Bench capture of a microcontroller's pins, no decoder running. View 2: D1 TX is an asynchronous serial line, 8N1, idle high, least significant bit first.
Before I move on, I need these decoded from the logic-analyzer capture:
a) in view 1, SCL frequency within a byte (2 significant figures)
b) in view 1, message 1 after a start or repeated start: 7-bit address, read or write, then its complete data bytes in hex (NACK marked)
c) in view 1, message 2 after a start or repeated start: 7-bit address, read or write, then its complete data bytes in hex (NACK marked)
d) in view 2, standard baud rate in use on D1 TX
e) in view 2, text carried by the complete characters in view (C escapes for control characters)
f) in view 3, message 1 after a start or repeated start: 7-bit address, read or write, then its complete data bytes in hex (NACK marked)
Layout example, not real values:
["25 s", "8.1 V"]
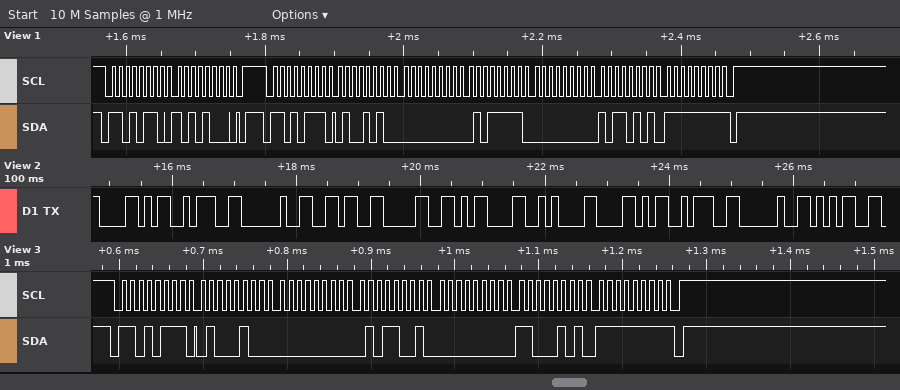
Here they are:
["100 kHz", "0x6B write: A8", "0x6B read: 4A 00 5F 00 B5 FF NACK", "9600 baud", "\"X: 60\\r\\nX: 5\"", "0x6B read: 44 00 59 00 C5 FF NACK"]
